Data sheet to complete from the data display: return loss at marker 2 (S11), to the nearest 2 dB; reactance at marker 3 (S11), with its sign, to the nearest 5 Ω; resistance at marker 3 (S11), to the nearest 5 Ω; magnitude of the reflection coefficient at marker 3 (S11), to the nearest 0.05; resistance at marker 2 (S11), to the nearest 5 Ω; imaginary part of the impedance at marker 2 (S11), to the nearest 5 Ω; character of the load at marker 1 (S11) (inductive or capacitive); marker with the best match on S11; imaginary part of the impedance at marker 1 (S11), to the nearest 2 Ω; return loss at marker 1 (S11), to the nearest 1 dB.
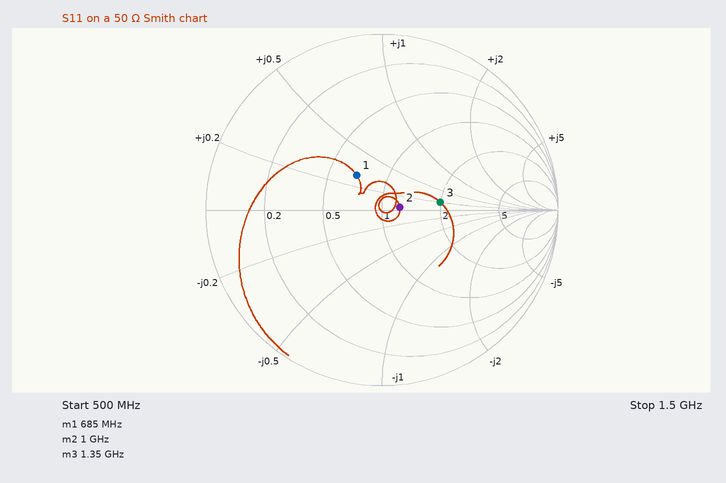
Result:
20 dB
+10 Ω
100 Ω
0.35
60 Ω
0 Ω
inductive
marker 2
+14 Ω
12 dB
